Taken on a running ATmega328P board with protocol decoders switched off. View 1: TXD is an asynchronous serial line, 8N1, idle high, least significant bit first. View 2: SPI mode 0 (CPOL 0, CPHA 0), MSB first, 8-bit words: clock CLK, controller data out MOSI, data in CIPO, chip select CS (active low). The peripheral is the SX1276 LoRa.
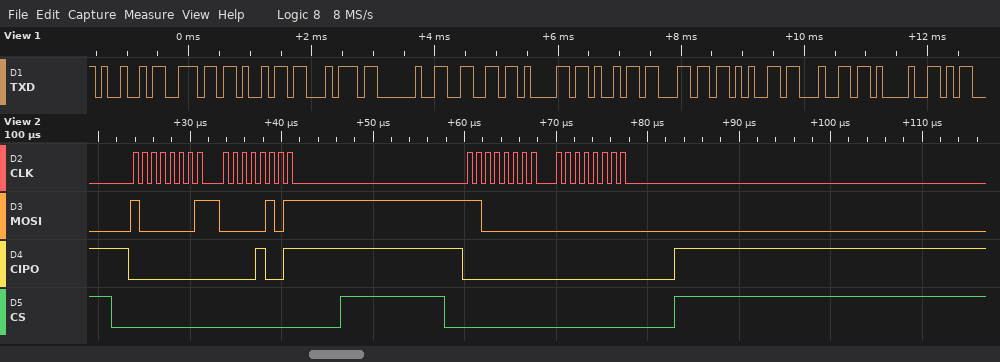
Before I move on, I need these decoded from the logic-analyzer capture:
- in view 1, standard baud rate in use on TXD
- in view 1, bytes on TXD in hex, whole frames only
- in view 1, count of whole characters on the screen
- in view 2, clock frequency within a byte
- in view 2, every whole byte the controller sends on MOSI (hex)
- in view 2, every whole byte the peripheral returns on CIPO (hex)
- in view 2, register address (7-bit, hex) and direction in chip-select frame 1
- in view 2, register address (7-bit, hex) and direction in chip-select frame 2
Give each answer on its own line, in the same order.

9600 baud
49 6E 69 74 20 66 61 69 6C 65 64 21
12
1 MHz
81 05 C0 00
00 09 00 00
0x01 write
0x40 write
